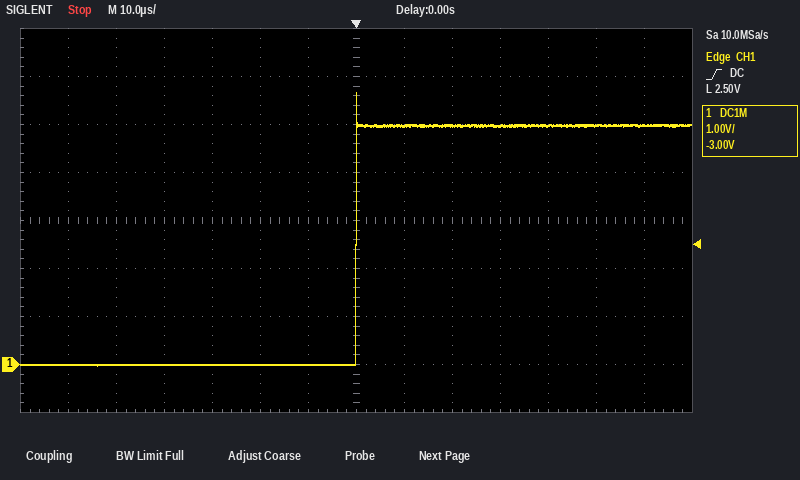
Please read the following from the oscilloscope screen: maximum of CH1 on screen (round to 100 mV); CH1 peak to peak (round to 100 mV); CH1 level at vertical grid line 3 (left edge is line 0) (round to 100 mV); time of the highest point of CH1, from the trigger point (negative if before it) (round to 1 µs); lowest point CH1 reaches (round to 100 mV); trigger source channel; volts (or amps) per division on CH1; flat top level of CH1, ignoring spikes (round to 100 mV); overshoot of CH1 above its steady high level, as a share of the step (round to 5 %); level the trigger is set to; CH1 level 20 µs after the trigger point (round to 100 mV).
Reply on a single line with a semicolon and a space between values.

5.7 V; 5.7 V; 0.0 V; 0 µs; 0.0 V; CH1; 1 V; 5.0 V; 15 %; 2.50 V; 5.0 V
